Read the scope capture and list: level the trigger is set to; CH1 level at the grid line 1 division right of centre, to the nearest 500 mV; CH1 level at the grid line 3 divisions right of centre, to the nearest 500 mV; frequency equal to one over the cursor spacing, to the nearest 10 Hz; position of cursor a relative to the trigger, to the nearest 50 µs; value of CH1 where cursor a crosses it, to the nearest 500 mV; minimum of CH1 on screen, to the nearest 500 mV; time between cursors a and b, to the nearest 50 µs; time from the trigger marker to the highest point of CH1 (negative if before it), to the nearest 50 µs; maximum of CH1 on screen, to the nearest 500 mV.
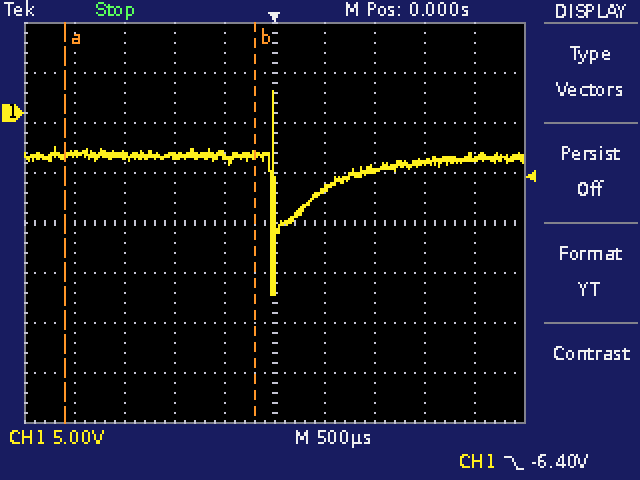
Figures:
-6.40 V
-7.5 V
-5.0 V
530 Hz
-2.10 ms
-4.0 V
-18.0 V
1.90 ms
0 µs
2.0 V
